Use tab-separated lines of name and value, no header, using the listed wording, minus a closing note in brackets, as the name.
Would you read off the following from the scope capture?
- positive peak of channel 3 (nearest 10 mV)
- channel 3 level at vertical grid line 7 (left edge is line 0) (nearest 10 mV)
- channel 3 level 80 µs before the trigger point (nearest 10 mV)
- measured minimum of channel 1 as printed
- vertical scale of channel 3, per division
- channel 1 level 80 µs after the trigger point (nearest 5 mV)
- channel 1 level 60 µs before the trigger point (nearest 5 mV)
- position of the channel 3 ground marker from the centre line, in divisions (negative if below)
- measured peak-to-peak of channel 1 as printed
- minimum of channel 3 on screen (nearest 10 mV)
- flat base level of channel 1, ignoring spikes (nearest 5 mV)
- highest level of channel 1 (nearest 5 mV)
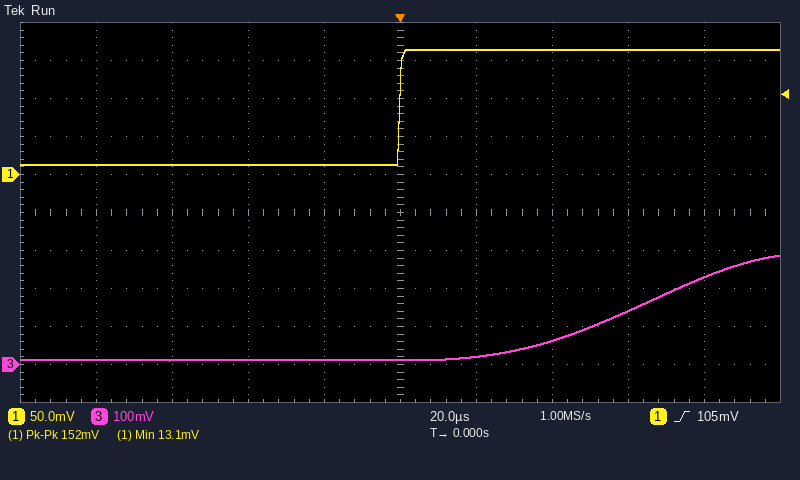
positive peak of channel 3	290 mV
channel 3 level at vertical grid line 7 (left edge is line 0)	60 mV
channel 3 level 80 µs before the trigger point	10 mV
measured minimum of channel 1 as printed	13.1 mV
vertical scale of channel 3, per division	100 mV
channel 1 level 80 µs after the trigger point	165 mV
channel 1 level 60 µs before the trigger point	15 mV
position of the channel 3 ground marker from the centre line, in divisions	-4.0 div
measured peak-to-peak of channel 1 as printed	152 mV
minimum of channel 3 on screen	10 mV
flat base level of channel 1, ignoring spikes	15 mV
highest level of channel 1	165 mV
